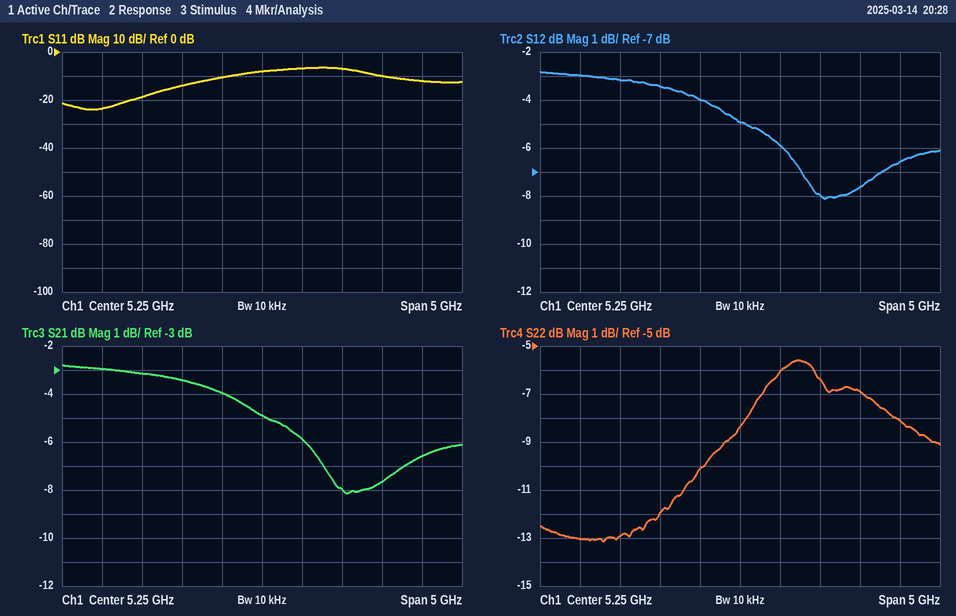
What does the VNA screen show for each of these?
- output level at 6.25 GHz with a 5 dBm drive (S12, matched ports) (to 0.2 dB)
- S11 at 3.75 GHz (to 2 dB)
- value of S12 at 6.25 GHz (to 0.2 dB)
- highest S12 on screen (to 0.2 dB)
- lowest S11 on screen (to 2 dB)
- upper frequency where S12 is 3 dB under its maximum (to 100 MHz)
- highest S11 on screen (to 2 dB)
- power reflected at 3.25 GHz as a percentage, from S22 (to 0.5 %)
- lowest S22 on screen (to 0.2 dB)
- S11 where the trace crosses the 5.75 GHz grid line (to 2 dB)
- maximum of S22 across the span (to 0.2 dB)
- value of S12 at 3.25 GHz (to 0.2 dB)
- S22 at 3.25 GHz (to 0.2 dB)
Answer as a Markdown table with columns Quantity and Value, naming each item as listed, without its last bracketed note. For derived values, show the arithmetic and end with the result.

| Quantity | Value |
|---|---|
| output level at 6.25 GHz with a 5 dBm drive (S12, matched ports) | 5 dBm + (-8.0 dB) = -3.0 dBm |
| S11 at 3.75 GHz | -18 dB |
| value of S12 at 6.25 GHz | -8.0 dB |
| highest S12 on screen | -2.8 dB |
| lowest S11 on screen | -24 dB |
| upper frequency where S12 is 3 dB under its maximum | 5.7 GHz |
| highest S11 on screen | -6 dB |
| power reflected at 3.25 GHz as a percentage, from S22 | 10^(-13/10) ≈ 5.0 % |
| lowest S22 on screen | -13.2 dB |
| S11 where the trace crosses the 5.75 GHz grid line | -6 dB |
| maximum of S22 across the span | -5.6 dB |
| value of S12 at 3.25 GHz | -3.0 dB |
| S22 at 3.25 GHz | -13.0 dB |
